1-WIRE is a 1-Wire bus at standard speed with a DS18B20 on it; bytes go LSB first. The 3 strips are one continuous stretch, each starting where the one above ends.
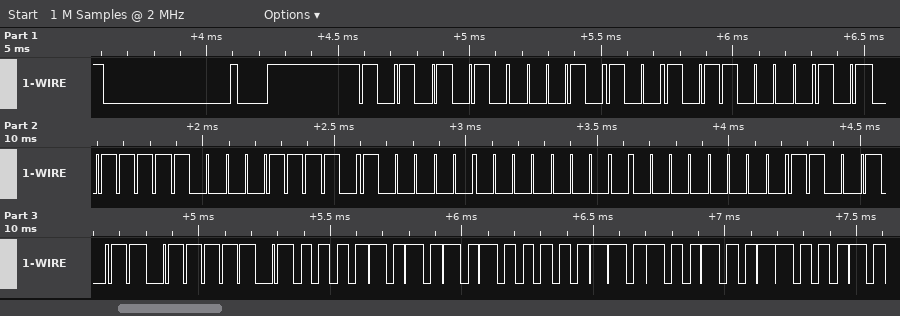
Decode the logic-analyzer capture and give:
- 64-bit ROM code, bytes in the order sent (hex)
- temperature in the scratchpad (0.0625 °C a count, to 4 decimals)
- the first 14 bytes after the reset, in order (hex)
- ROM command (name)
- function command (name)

28 0D F5 E1 05 00 00 D3
85.0000 °C
55 28 0D F5 E1 05 00 00 D3 BE 50 05 4B 46
Match ROM
Read Scratchpad
